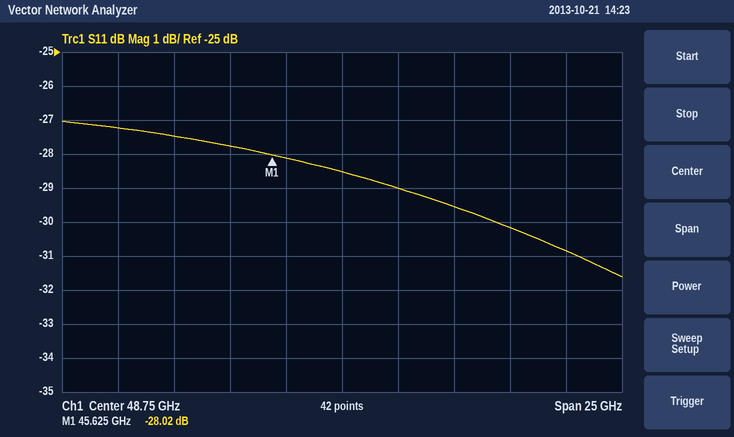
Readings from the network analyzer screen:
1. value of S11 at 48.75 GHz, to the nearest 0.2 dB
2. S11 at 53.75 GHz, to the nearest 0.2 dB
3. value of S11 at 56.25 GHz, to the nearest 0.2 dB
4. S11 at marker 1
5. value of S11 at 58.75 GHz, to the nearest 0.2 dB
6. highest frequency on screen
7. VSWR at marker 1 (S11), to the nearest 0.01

-28.6 dB
-29.6 dB
-30.2 dB
-28.02 dB
-30.8 dB
61.25 GHz
1.08
